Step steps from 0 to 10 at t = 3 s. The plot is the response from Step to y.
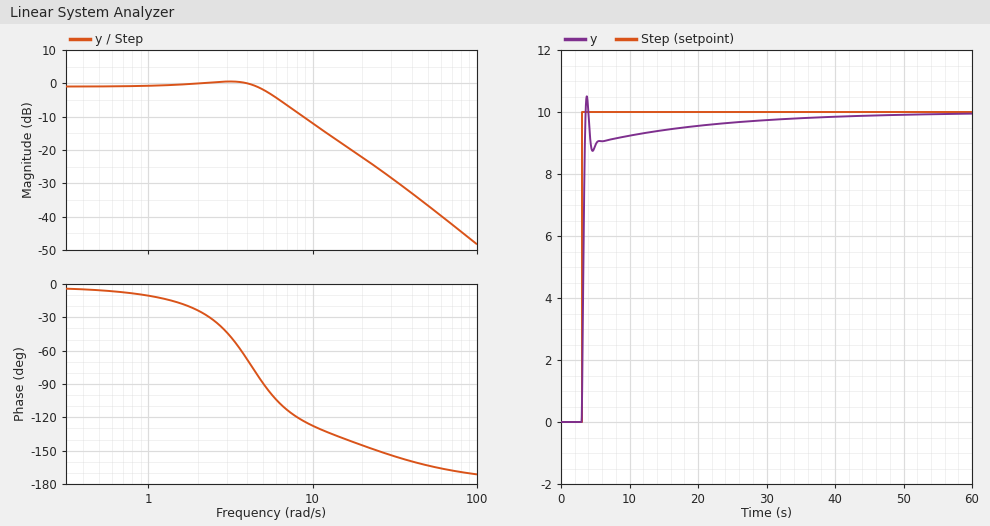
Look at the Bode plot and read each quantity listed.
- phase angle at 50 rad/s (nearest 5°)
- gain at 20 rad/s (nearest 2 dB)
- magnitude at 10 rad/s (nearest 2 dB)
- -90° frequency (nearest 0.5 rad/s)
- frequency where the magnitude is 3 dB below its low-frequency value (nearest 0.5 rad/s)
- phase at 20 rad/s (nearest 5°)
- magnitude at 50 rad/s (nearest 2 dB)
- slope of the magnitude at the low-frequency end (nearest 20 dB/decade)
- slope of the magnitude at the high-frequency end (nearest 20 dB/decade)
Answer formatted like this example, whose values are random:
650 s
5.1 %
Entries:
-165°
-22 dB
-12 dB
5.0 rad/s
6.0 rad/s
-145°
-36 dB
0 dB/decade
-40 dB/decade
